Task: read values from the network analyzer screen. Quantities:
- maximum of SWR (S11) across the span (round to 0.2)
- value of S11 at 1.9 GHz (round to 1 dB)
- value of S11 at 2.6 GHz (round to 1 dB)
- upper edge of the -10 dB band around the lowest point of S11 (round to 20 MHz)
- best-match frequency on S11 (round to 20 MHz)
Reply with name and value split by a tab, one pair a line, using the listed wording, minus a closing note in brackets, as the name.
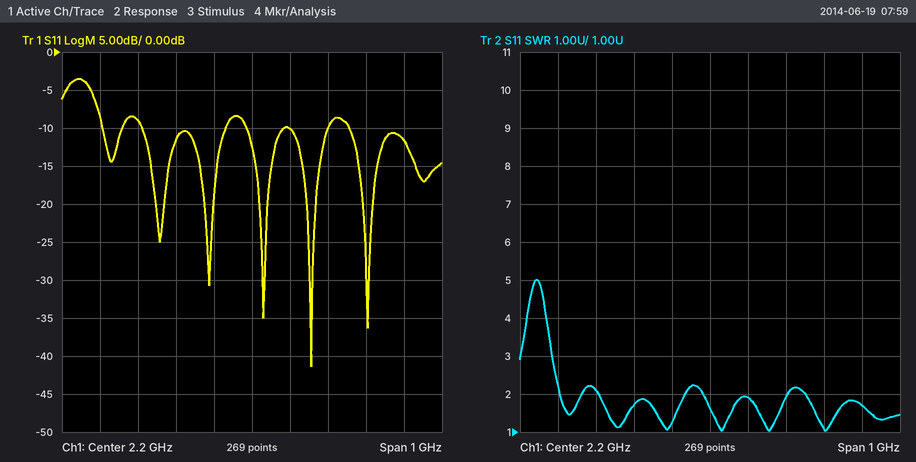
maximum of SWR (S11) across the span	5.0
value of S11 at 1.9 GHz	-9 dB
value of S11 at 2.6 GHz	-12 dB
upper edge of the -10 dB band around the lowest point of S11	2.40 GHz
best-match frequency on S11	2.36 GHz
